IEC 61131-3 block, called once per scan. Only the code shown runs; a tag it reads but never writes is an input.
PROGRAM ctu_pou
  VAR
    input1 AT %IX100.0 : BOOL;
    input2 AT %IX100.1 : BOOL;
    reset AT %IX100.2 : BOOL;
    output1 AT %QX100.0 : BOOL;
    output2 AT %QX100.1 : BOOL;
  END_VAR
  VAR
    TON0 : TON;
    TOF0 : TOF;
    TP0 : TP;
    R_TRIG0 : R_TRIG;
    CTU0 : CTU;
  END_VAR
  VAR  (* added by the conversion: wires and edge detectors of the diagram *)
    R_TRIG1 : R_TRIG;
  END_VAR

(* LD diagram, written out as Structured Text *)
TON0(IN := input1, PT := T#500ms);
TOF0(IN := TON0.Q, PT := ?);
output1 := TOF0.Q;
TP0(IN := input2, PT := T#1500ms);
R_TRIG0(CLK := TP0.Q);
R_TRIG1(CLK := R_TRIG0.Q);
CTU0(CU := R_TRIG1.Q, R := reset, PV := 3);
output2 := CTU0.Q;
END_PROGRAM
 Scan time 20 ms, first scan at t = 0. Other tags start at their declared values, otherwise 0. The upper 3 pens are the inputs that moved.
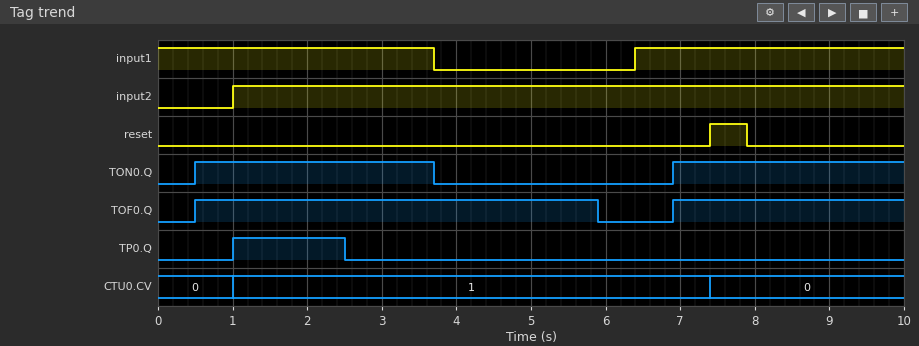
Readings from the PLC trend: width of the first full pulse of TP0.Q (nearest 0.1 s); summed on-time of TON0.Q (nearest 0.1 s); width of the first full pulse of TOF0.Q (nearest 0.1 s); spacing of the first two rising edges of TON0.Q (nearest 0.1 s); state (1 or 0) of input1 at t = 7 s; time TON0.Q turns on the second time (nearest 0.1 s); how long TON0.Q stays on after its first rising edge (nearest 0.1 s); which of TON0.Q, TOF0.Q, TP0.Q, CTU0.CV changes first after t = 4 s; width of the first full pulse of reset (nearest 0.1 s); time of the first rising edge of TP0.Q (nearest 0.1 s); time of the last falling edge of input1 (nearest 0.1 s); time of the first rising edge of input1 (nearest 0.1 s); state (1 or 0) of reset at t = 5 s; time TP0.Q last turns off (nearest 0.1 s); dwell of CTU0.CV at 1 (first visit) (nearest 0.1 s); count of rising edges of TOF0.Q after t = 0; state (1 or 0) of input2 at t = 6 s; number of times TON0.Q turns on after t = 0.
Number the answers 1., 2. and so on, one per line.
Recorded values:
1. 1.5 s
2. 6.3 s
3. 5.4 s
4. 6.4 s
5. 1
6. 6.9 s
7. 3.2 s
8. TOF0.Q
9. 0.5 s
10. 1.0 s
11. 3.7 s
12. 6.4 s
13. 0
14. 2.5 s
15. 6.4 s
16. 2
17. 1
18. 2
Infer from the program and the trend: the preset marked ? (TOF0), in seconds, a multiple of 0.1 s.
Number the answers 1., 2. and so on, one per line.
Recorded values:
1. 2.2 s
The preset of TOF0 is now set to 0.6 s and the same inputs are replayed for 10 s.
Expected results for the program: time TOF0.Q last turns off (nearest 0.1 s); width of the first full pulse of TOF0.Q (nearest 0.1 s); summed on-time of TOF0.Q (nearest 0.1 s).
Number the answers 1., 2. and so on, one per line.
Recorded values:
1. 4.3 s
2. 3.8 s
3. 6.9 s
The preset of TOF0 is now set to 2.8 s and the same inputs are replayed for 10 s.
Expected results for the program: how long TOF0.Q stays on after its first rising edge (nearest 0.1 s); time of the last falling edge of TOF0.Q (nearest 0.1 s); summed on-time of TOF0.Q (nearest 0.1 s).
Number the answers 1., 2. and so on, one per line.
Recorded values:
1. 6.0 s
2. 6.5 s
3. 9.1 s
